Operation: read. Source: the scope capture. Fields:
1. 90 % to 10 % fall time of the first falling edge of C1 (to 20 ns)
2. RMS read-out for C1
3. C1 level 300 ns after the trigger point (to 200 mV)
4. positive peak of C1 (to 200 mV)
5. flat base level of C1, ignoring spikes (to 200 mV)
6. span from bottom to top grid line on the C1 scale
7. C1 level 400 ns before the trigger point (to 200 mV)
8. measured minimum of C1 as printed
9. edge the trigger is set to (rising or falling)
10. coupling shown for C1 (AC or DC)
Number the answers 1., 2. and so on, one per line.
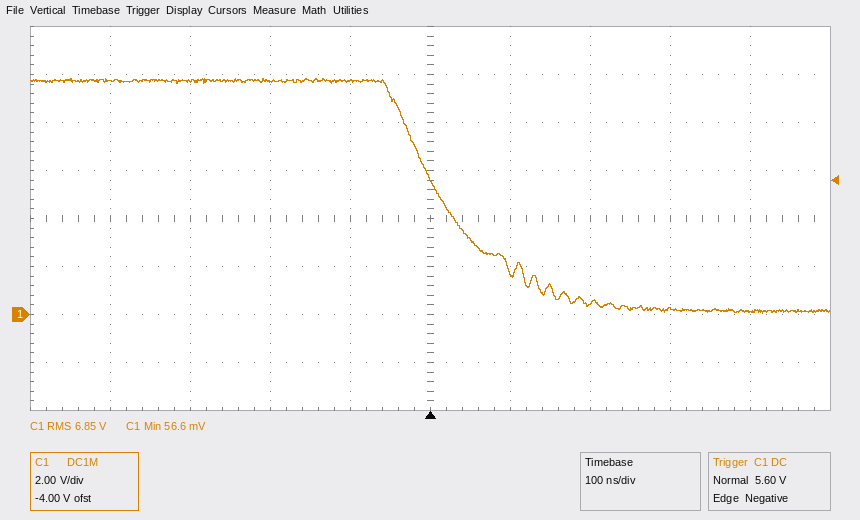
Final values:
1. 180 ns
2. 6.85 V
3. 200 mV
4. 9.8 V
5. 200 mV
6. 16 V
7. 9.8 V
8. 56.6 mV
9. falling
10. DC
